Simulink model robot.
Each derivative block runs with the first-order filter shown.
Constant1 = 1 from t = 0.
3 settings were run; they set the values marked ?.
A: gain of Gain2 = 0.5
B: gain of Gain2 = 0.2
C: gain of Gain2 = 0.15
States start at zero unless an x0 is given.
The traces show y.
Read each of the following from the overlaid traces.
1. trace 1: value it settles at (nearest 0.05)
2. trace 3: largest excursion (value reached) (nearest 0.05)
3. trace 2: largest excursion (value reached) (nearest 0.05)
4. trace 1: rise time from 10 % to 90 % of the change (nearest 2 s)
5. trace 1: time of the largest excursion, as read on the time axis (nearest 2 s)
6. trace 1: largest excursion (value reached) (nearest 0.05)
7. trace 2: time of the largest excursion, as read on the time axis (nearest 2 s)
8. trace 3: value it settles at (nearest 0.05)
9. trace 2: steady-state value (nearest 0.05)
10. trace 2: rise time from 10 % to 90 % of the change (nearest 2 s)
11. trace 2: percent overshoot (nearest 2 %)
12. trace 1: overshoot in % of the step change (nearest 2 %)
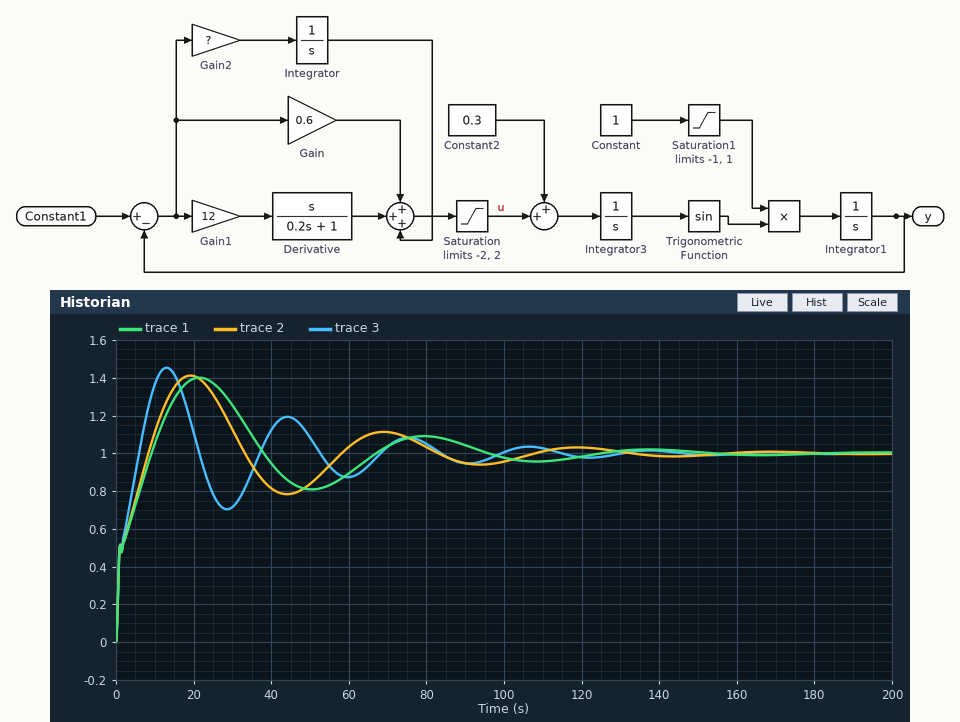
1.00
1.45
1.40
8 s
22 s
1.40
20 s
1.00
1.00
6 s
42 %
40 %
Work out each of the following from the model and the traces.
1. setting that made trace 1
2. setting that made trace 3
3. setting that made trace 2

C
A
B
